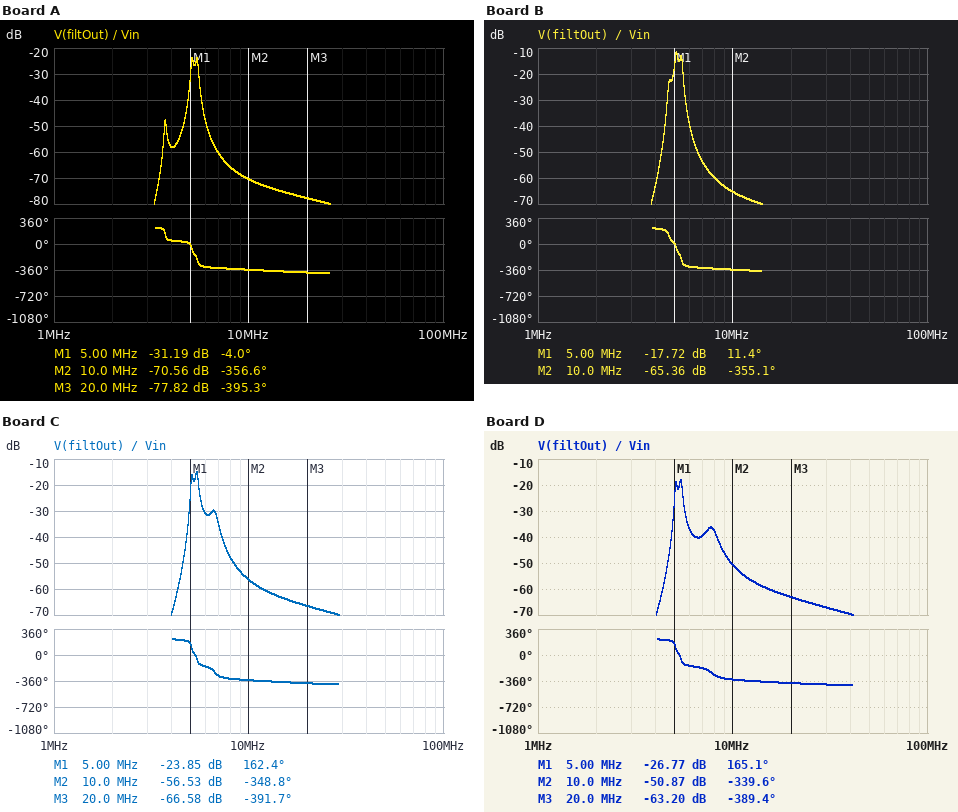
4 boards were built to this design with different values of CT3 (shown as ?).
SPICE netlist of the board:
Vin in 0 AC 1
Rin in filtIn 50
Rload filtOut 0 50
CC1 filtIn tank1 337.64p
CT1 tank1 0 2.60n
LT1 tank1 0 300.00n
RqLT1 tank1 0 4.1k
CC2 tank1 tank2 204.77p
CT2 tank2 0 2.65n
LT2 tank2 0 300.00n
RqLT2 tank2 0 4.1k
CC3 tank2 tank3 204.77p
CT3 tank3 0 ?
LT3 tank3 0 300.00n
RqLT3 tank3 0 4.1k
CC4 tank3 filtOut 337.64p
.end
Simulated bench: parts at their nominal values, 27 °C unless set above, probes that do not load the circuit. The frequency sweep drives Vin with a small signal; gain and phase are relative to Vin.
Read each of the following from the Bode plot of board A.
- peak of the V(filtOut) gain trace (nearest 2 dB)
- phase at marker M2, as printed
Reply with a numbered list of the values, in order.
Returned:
1. -24 dB
2. -356.6 deg
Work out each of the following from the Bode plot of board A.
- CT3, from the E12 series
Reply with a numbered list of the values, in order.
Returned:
1. 5.6 nF
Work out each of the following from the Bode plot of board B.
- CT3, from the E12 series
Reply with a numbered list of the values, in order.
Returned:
1. 3.3 nF
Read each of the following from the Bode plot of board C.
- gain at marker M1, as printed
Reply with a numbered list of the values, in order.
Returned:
1. -23.85 dB
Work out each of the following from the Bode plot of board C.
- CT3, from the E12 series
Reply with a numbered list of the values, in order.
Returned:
1. 1.5 nF
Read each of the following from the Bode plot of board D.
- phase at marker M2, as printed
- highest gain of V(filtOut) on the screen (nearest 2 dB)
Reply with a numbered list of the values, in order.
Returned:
1. -339.6 deg
2. -18 dB
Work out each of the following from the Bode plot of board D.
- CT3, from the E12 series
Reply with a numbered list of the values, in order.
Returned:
1. 1 nF
